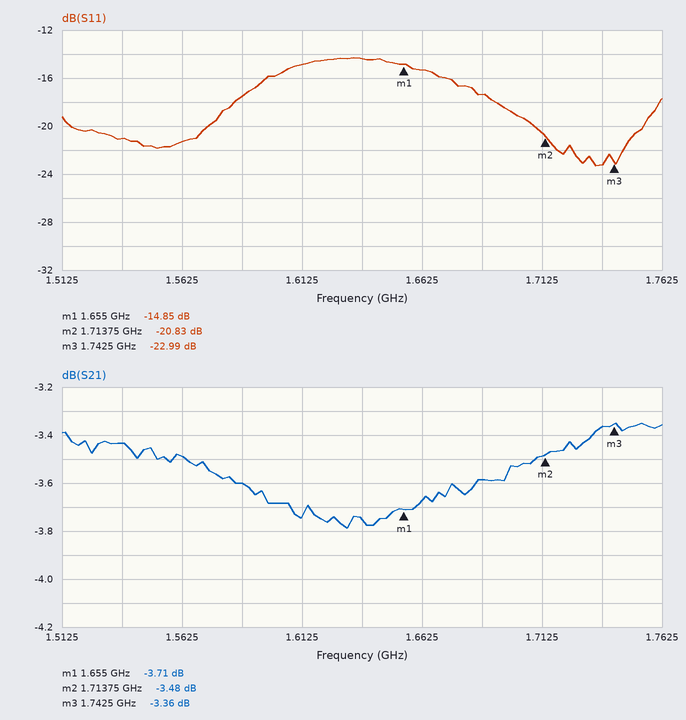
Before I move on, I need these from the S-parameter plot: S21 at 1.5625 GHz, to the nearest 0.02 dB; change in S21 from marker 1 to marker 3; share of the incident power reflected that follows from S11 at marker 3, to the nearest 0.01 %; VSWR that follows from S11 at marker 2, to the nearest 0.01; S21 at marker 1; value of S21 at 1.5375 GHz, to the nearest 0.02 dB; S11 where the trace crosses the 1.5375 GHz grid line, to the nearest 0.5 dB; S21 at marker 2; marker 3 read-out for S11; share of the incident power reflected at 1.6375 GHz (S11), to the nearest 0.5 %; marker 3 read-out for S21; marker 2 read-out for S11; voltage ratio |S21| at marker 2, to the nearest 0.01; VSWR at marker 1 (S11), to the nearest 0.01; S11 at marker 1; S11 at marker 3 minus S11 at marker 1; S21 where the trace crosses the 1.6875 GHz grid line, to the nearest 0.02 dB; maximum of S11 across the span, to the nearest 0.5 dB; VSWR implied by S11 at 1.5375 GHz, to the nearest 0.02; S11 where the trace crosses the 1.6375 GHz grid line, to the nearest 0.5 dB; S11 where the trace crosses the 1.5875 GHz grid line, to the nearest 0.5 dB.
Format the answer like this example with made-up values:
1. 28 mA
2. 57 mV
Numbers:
1. -3.48 dB
2. 0.35 dB
3. 0.50 %
4. 1.20
5. -3.71 dB
6. -3.44 dB
7. -21.0 dB
8. -3.48 dB
9. -22.99 dB
10. 3.5 %
11. -3.36 dB
12. -20.83 dB
13. 0.67
14. 1.44
15. -14.85 dB
16. -8.14 dB
17. -3.58 dB
18. -14.5 dB
19. 1.20
20. -14.5 dB
21. -17.5 dB
